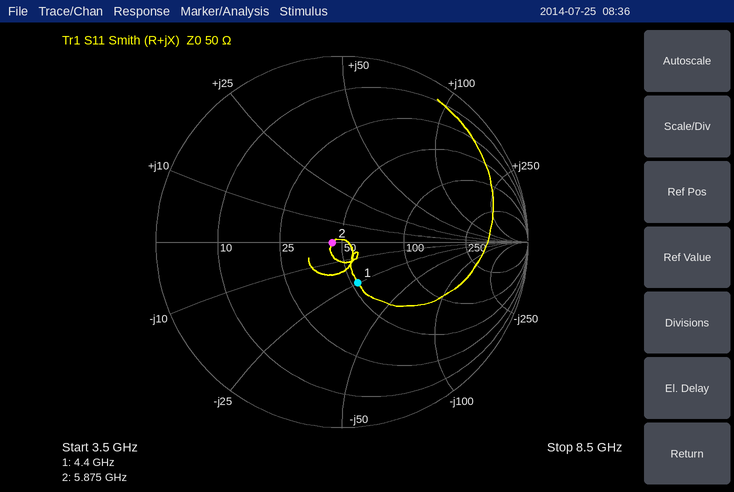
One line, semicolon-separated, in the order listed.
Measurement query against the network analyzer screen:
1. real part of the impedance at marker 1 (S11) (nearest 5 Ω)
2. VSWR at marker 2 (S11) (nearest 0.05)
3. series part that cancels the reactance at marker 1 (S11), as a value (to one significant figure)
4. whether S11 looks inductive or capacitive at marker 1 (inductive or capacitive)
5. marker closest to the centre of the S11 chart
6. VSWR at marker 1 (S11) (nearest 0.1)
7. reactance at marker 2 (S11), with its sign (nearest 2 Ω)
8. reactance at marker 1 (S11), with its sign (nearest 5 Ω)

55 Ω; 1.10; 900 pH; capacitive; marker 2; 1.6; 0 Ω; -25 Ω
